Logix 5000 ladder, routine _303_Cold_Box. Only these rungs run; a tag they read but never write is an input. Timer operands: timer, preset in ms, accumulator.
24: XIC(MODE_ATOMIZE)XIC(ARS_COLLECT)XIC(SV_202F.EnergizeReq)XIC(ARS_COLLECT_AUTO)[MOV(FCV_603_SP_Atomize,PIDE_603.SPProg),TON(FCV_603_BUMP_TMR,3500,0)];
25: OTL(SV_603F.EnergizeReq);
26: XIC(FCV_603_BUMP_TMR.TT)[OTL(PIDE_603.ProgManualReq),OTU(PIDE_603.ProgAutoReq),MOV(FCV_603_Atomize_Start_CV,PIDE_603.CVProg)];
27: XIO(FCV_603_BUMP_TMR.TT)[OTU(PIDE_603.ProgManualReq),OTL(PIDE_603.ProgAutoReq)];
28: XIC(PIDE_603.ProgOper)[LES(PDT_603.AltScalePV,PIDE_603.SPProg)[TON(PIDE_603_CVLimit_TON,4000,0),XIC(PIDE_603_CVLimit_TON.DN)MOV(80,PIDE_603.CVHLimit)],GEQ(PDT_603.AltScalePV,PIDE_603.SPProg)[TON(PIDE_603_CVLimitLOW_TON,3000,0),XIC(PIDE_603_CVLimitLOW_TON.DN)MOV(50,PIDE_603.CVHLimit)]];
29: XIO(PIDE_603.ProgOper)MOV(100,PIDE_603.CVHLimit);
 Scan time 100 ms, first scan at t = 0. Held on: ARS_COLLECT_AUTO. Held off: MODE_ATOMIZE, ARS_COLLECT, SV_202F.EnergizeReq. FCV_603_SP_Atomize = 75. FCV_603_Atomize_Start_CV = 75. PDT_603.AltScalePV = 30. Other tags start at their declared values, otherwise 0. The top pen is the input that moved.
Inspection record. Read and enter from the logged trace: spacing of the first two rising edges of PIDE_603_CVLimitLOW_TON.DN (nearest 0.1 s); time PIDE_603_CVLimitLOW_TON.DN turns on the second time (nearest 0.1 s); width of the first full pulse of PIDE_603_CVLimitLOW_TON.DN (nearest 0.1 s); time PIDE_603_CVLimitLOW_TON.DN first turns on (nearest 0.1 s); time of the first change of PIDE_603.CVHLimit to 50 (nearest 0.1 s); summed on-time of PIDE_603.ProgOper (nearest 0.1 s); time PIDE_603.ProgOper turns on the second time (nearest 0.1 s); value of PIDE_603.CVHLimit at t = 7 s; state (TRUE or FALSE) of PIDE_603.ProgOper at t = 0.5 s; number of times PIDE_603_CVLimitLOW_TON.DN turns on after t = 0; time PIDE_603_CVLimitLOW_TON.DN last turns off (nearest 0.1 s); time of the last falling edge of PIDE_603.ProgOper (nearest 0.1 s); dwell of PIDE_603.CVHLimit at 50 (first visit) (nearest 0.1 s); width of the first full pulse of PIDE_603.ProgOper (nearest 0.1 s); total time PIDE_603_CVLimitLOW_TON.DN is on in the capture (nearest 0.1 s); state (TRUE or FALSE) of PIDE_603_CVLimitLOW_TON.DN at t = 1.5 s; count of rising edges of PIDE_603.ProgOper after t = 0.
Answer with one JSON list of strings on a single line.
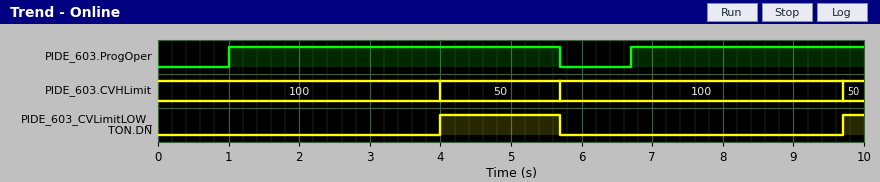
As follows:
["5.7 s", "9.7 s", "1.7 s", "4.0 s", "4.0 s", "8.0 s", "6.7 s", "100", "FALSE", "2", "5.7 s", "5.7 s", "1.7 s", "4.7 s", "2.0 s", "FALSE", "2"]
